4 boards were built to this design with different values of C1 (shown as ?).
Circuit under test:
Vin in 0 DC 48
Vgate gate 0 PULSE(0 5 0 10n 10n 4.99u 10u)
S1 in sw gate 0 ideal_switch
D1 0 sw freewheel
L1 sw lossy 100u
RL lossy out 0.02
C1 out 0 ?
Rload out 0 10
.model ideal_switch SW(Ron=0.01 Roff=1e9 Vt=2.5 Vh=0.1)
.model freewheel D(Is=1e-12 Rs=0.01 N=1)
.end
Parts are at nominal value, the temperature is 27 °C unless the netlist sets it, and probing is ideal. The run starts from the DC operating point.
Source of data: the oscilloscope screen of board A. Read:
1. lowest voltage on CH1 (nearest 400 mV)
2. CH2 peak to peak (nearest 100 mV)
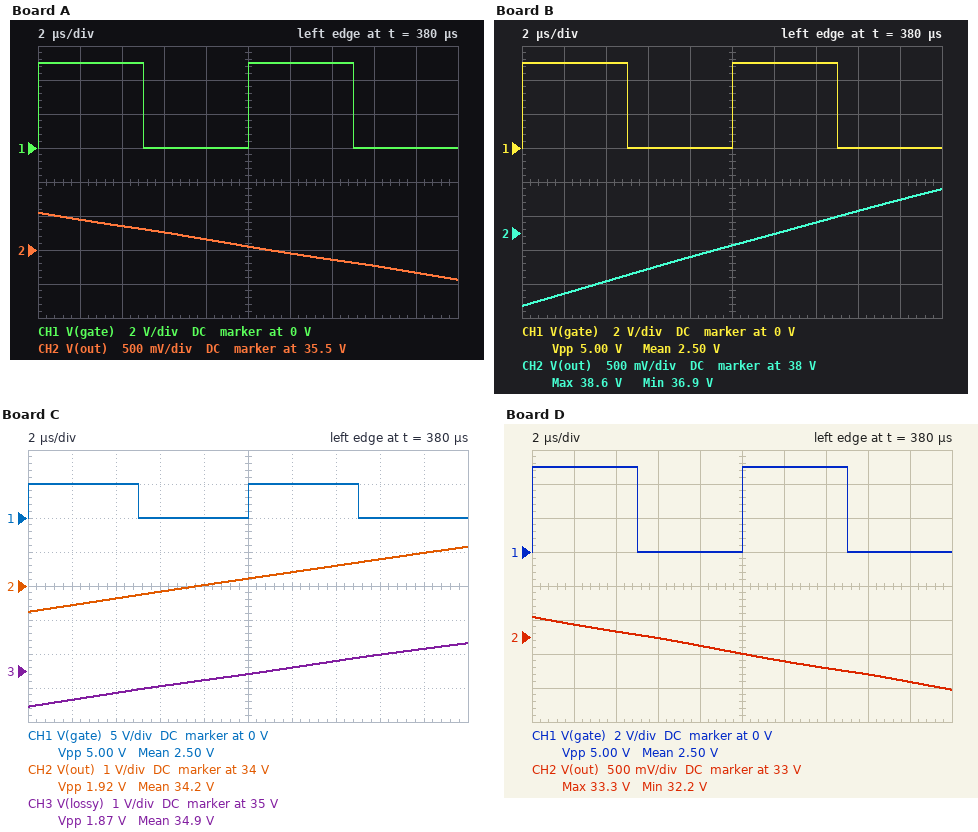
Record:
0 V
1.0 V
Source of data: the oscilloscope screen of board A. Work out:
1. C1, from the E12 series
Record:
68 µF
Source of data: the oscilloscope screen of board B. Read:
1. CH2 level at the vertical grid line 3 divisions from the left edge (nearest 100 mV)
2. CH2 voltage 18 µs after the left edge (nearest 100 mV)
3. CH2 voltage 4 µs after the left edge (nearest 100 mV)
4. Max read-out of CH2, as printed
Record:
37.5 V
38.5 V
37.3 V
38.6 V
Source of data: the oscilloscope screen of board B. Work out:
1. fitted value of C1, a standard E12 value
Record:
270 µF
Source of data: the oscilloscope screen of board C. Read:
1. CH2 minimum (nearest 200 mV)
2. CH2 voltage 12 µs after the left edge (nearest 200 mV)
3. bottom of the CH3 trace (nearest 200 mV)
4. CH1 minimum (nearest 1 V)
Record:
33.2 V
34.4 V
34.0 V
0 V
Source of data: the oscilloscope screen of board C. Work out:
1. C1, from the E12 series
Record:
330 µF
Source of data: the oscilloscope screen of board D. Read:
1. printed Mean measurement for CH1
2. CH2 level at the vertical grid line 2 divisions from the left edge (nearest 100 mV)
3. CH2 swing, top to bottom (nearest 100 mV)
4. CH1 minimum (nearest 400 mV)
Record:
2.50 V
33.1 V
1.1 V
0 V
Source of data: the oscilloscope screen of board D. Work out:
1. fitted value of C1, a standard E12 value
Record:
56 µF
